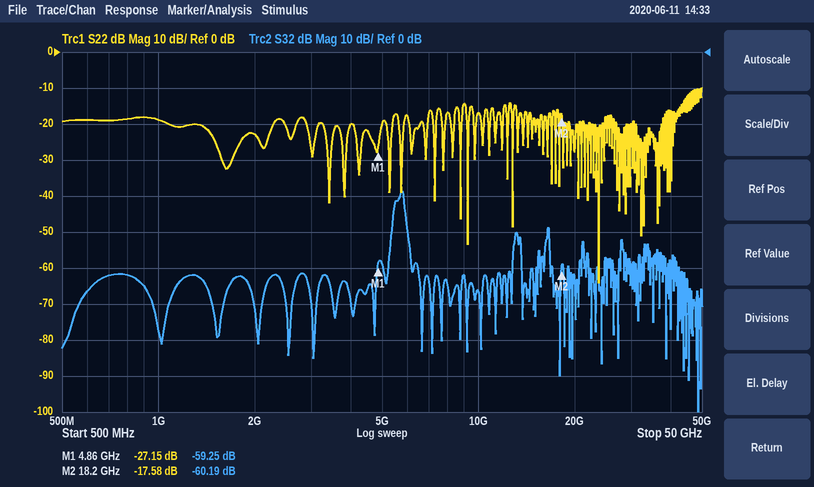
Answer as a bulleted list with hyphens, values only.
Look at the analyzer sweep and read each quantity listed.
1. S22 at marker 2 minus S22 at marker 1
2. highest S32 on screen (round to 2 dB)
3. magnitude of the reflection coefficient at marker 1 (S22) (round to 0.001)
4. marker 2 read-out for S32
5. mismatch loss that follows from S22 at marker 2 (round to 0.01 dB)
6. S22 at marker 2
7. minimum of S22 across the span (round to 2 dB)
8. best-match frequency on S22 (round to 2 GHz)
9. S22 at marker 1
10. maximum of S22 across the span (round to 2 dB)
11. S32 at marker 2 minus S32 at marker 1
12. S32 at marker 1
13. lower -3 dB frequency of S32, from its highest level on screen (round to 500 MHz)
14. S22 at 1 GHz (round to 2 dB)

- 9.57 dB
- -38 dB
- 0.044
- -60.19 dB
- 0.08 dB
- -17.58 dB
- -64 dB
- 24 GHz
- -27.15 dB
- -10 dB
- -0.94 dB
- -59.25 dB
- 5.5 GHz
- -18 dB
